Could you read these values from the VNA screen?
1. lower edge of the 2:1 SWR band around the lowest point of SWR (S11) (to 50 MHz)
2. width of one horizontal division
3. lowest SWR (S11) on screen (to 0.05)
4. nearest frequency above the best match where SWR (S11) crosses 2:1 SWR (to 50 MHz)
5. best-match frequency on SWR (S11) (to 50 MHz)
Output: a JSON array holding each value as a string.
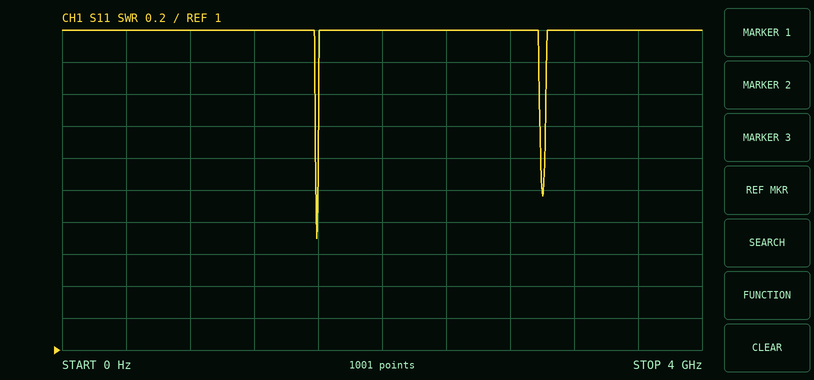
["1.60 GHz", "400 MHz", "1.70", "1.60 GHz", "1.60 GHz"]
